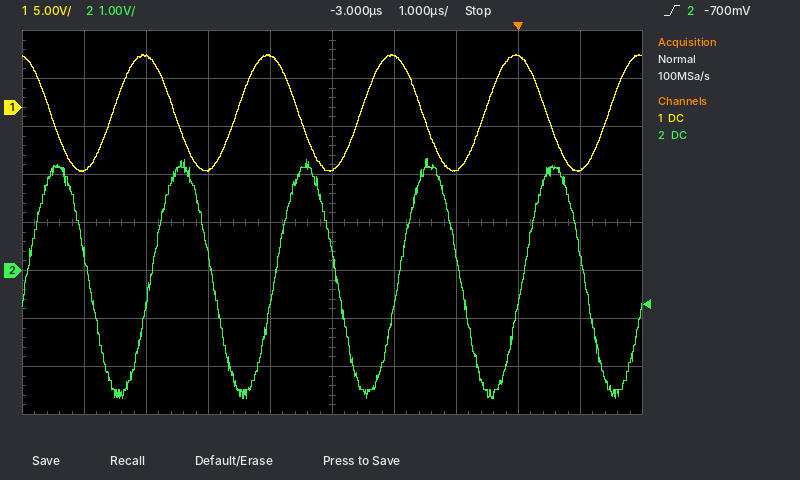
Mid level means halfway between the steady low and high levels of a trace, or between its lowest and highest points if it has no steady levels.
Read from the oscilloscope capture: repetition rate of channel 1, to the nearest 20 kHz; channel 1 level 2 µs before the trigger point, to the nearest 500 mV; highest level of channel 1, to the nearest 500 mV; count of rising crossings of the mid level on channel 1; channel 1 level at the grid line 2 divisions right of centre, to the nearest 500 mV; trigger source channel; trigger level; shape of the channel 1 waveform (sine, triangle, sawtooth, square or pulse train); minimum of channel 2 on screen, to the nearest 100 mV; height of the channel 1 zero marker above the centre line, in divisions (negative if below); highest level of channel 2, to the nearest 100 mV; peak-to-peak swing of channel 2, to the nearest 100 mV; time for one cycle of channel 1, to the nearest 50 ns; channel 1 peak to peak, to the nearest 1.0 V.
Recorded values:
500 kHz
5.5 V
5.5 V
5
-6.5 V
channel 2
-700 mV
sine
-2.7 V
+2.4 div
2.3 V
5.0 V
2.00 µs
12.0 V
